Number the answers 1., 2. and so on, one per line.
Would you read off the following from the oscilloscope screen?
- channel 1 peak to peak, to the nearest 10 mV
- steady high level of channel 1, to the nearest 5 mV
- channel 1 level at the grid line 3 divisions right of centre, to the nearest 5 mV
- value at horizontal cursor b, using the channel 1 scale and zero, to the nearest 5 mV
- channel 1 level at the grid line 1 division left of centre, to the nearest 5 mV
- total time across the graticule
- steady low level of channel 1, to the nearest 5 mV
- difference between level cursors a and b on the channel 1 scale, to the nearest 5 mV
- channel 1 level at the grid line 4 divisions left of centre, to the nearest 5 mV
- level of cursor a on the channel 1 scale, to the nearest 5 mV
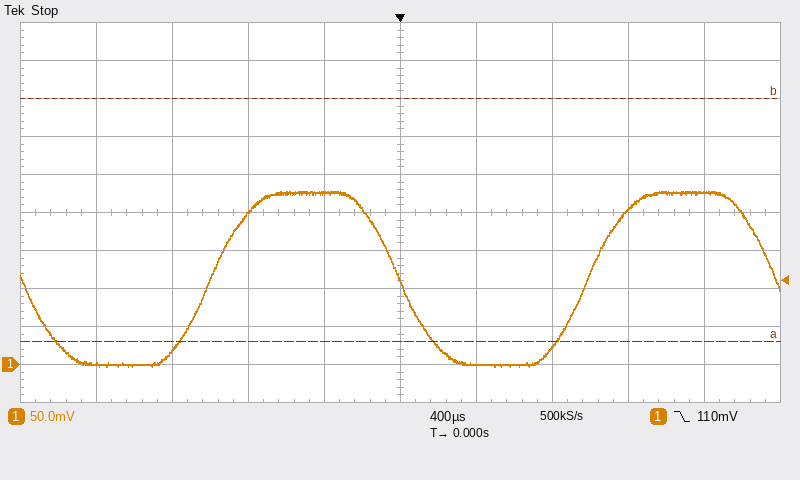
1. 230 mV
2. 225 mV
3. 205 mV
4. 350 mV
5. 225 mV
6. 4 ms
7. 0 mV
8. 320 mV
9. 0 mV
10. 30 mV
